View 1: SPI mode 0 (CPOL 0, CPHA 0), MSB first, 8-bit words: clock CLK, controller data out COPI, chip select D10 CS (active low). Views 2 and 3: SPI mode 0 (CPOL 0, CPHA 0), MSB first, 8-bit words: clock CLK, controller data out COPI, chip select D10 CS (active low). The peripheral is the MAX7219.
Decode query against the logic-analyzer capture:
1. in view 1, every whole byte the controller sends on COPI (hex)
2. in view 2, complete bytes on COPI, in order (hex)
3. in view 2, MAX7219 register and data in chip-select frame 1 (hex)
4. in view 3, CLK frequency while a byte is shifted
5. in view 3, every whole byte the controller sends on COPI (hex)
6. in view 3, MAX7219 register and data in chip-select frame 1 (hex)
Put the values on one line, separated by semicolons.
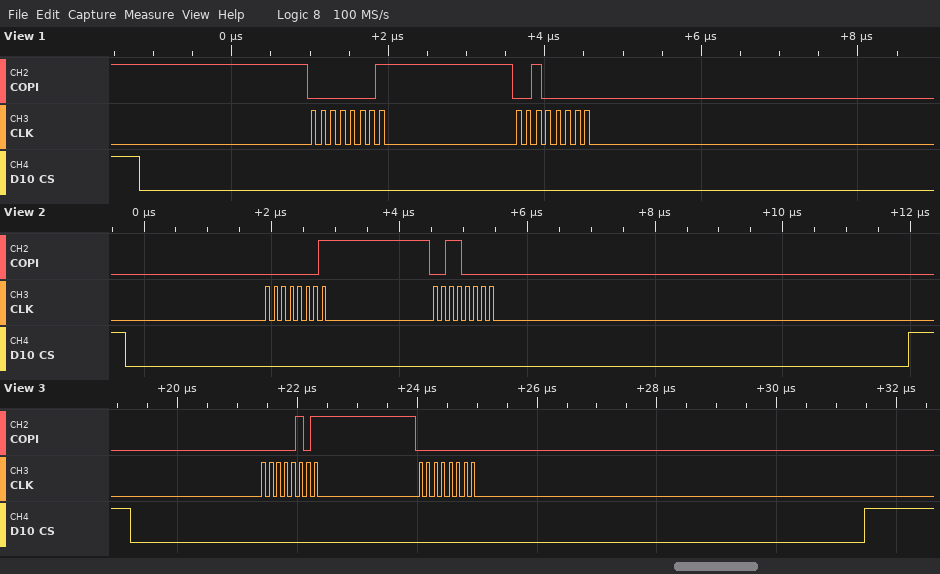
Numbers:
0x01 0x20; 01 30; register 0x1, data 0x30; 8 MHz; 0x05 0x00; register 0x5, data 0x00
